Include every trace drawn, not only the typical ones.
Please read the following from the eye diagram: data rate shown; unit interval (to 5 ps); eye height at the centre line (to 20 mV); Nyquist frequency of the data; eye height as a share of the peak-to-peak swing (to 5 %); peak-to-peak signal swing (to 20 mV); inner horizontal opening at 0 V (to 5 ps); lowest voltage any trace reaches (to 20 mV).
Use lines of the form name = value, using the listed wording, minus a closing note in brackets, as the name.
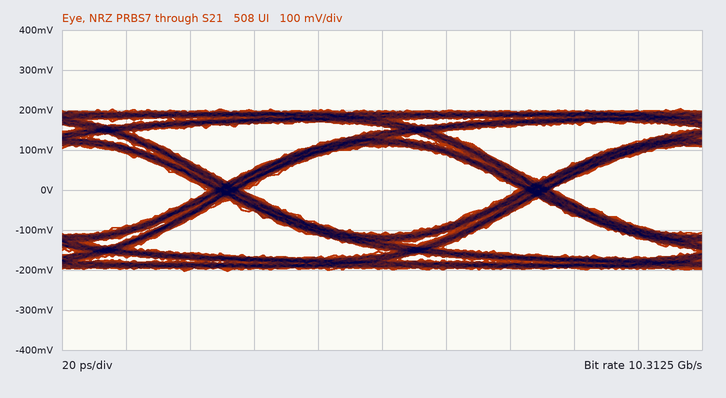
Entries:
data rate shown = 10.3125 Gb/s
unit interval = 95 ps
eye height at the centre line = 220 mV
Nyquist frequency of the data = 5.15625 GHz
eye height as a share of the peak-to-peak swing = 55 %
peak-to-peak signal swing = 400 mV
inner horizontal opening at 0 V = 85 ps
lowest voltage any trace reaches = -200 mV
